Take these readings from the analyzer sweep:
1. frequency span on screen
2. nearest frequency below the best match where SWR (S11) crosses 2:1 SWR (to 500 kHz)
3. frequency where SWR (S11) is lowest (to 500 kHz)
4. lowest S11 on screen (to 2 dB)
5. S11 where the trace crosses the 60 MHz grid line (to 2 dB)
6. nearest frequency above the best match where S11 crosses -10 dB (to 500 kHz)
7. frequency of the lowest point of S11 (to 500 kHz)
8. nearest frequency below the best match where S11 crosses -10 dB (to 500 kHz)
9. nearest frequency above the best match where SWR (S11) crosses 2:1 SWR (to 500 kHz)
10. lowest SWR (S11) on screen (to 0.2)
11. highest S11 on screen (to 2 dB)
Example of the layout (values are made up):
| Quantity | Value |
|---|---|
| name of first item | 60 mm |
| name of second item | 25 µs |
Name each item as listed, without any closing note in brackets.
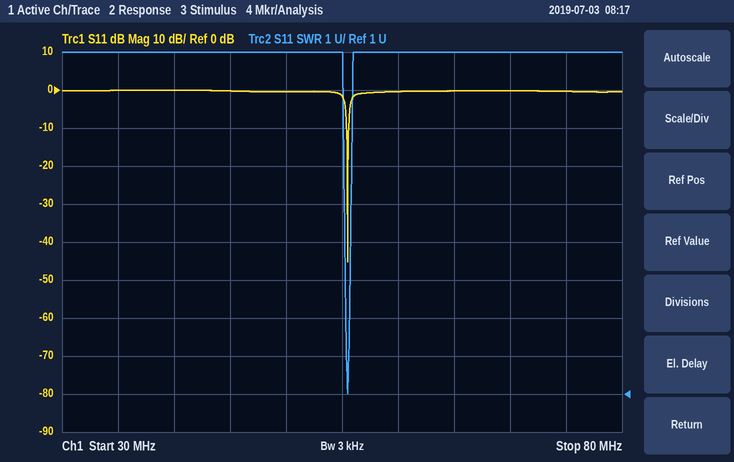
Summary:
| Quantity | Value |
|---|---|
| frequency span on screen | 50 MHz |
| nearest frequency below the best match where SWR (S11) crosses 2:1 SWR | 55.5 MHz |
| frequency where SWR (S11) is lowest | 55.5 MHz |
| lowest S11 on screen | -46 dB |
| S11 where the trace crosses the 60 MHz grid line | 0 dB |
| nearest frequency above the best match where S11 crosses -10 dB | 55.5 MHz |
| frequency of the lowest point of S11 | 55.5 MHz |
| nearest frequency below the best match where S11 crosses -10 dB | 55.5 MHz |
| nearest frequency above the best match where SWR (S11) crosses 2:1 SWR | 55.5 MHz |
| lowest SWR (S11) on screen | 1.0 |
| highest S11 on screen | 0 dB |
